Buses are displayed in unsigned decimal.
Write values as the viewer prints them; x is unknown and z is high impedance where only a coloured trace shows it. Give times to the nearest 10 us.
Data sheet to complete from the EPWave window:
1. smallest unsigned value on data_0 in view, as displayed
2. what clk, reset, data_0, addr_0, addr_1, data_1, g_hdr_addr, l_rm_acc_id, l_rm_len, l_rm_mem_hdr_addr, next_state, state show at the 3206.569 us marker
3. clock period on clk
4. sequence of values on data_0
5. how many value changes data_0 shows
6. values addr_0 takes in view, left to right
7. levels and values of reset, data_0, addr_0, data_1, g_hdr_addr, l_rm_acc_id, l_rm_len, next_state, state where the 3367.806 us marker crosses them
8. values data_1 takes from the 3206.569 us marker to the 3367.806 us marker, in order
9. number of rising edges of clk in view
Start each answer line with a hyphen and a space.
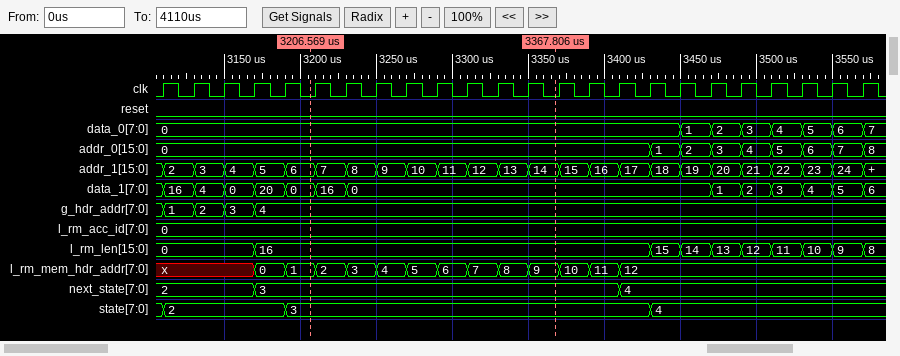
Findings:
- 0
- clk=0, reset=0, data_0=0, addr_0=0, addr_1=6, data_1=0, g_hdr_addr=4, l_rm_acc_id=0, l_rm_len=16, l_rm_mem_hdr_addr=1, next_state=3, state=3
- 20 us
- 0, 1, 2, 3, 4, 5, 6, 7
- 7
- 0, 1, 2, 3, 4, 5, 6, 7, 8
- reset=0, data_0=0, addr_0=0, data_1=0, g_hdr_addr=4, l_rm_acc_id=0, l_rm_len=16, next_state=3, state=3
- 0, 16, 0
- 24
